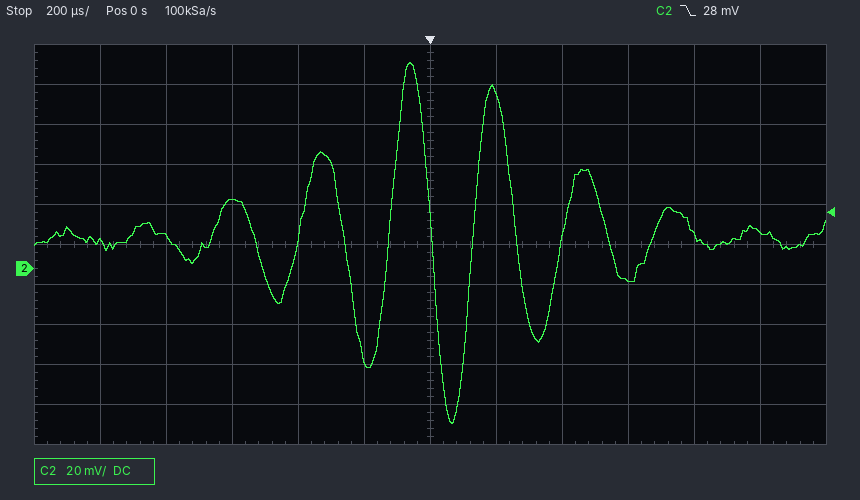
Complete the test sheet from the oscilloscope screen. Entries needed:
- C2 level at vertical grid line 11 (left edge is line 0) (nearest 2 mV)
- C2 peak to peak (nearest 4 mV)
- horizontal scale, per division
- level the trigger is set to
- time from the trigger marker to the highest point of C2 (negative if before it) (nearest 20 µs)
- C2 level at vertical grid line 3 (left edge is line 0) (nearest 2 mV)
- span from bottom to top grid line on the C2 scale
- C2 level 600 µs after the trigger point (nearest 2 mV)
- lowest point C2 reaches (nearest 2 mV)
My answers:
18 mV
180 mV
200 µs
28 mV
-60 µs
34 mV
200 mV
-6 mV
-78 mV
